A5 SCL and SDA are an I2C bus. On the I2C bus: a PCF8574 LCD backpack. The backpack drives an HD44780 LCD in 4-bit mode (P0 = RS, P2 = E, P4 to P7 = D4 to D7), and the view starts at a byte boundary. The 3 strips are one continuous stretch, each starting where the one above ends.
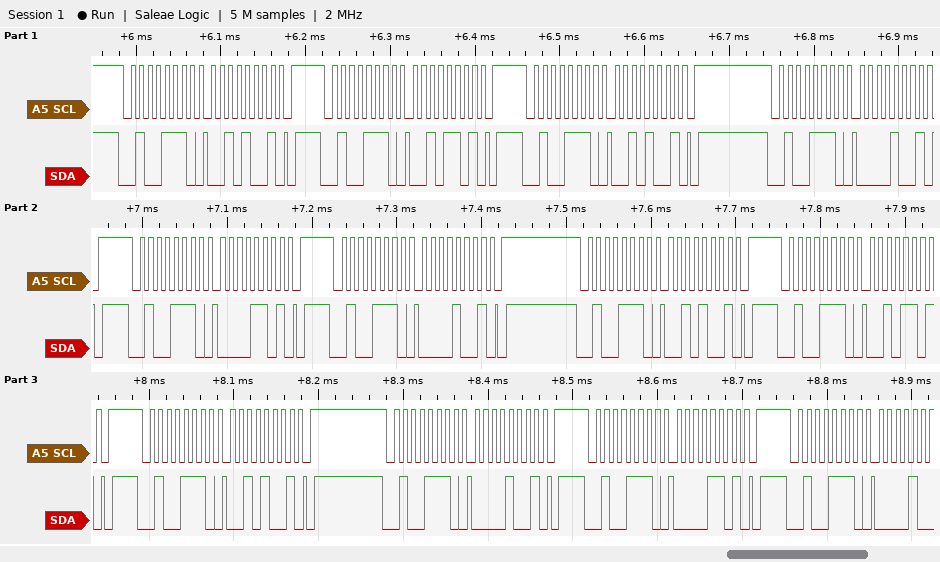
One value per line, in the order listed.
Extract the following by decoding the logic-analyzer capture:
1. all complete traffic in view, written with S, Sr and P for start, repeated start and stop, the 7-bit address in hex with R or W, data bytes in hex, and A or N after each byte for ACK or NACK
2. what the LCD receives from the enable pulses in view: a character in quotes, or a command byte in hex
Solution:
S 27W A 29 A P S 27W A 2D A P S 27W A 29 A P S 27W A 09 A P S 27W A 0D A P S 27W A 09 A P S 27W A 29 A P S 27W A 2D A P S 27W A 29 A P S 27W A 09 A P S 27W A 0D A P S 27W A
' '
